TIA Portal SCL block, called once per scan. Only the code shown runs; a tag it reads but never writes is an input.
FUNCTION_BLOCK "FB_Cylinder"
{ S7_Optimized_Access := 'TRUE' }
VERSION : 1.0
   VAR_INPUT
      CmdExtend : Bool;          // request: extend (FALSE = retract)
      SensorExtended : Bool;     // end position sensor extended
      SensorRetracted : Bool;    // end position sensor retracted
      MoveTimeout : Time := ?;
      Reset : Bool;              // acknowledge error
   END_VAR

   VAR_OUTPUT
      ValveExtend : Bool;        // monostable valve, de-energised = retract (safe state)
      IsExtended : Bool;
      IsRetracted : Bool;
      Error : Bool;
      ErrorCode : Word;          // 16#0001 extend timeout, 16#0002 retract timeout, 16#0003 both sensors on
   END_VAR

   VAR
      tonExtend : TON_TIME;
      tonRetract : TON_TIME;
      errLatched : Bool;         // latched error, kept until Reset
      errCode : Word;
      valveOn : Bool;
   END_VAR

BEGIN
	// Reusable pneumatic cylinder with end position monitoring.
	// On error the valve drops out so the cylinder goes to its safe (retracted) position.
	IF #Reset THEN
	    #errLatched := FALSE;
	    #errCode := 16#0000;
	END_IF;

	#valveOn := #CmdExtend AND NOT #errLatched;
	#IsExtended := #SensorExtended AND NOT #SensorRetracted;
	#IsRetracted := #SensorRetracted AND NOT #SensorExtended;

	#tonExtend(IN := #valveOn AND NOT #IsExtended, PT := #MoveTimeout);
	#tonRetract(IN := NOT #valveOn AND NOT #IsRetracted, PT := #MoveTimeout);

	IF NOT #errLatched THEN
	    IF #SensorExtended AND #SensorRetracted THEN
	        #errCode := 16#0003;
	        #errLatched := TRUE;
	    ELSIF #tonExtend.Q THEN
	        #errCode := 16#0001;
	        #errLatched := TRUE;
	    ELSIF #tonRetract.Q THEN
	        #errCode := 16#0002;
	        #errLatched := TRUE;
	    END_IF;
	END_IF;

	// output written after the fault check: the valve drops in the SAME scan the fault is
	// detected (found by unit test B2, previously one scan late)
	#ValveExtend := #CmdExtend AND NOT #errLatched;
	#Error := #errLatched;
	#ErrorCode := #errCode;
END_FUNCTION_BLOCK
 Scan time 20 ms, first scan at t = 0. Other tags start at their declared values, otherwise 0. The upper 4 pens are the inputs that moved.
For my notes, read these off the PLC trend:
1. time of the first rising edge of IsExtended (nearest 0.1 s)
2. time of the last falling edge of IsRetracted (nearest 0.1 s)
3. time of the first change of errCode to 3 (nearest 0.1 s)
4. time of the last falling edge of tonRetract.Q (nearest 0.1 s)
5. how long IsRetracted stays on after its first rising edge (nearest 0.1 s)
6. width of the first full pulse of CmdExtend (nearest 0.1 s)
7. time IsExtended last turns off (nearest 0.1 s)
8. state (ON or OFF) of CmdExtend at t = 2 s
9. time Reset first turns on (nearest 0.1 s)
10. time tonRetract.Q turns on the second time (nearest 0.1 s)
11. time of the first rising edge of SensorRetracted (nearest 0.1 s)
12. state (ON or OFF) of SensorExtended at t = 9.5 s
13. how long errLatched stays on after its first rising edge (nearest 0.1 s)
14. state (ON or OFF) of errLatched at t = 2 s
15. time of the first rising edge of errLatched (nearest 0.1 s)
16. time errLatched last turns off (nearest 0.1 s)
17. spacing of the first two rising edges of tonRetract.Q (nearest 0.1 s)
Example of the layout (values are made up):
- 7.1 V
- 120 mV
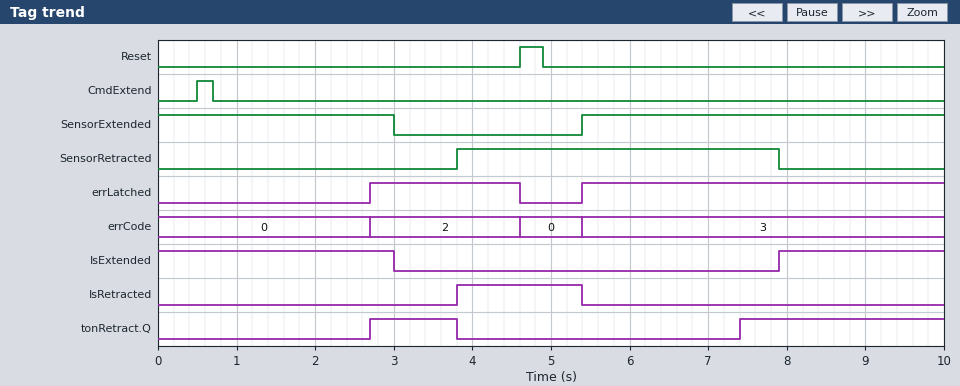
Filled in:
- 7.9 s
- 5.4 s
- 5.4 s
- 3.8 s
- 1.6 s
- 0.2 s
- 3.0 s
- OFF
- 4.6 s
- 7.4 s
- 3.8 s
- ON
- 1.9 s
- OFF
- 2.7 s
- 4.6 s
- 4.7 s
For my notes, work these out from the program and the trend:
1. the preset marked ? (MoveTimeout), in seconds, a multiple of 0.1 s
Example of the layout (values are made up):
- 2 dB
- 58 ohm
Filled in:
- 2.0 s
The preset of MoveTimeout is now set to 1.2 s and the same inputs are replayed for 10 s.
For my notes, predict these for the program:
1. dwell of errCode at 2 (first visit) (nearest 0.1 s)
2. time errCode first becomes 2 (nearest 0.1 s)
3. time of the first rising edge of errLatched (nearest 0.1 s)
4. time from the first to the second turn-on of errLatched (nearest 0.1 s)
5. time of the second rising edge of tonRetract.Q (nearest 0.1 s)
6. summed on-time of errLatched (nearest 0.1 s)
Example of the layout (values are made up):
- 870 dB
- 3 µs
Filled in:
- 2.7 s
- 1.9 s
- 1.9 s
- 3.5 s
- 6.6 s
- 7.3 s
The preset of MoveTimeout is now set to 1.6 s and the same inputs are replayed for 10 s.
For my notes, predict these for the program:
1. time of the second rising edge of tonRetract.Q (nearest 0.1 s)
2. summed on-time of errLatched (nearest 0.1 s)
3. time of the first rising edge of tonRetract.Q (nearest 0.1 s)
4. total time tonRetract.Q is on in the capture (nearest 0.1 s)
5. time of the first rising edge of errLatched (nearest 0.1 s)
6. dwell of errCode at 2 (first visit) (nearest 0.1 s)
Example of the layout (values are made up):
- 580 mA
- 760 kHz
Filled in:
- 7.0 s
- 6.9 s
- 2.3 s
- 4.5 s
- 2.3 s
- 2.3 s
